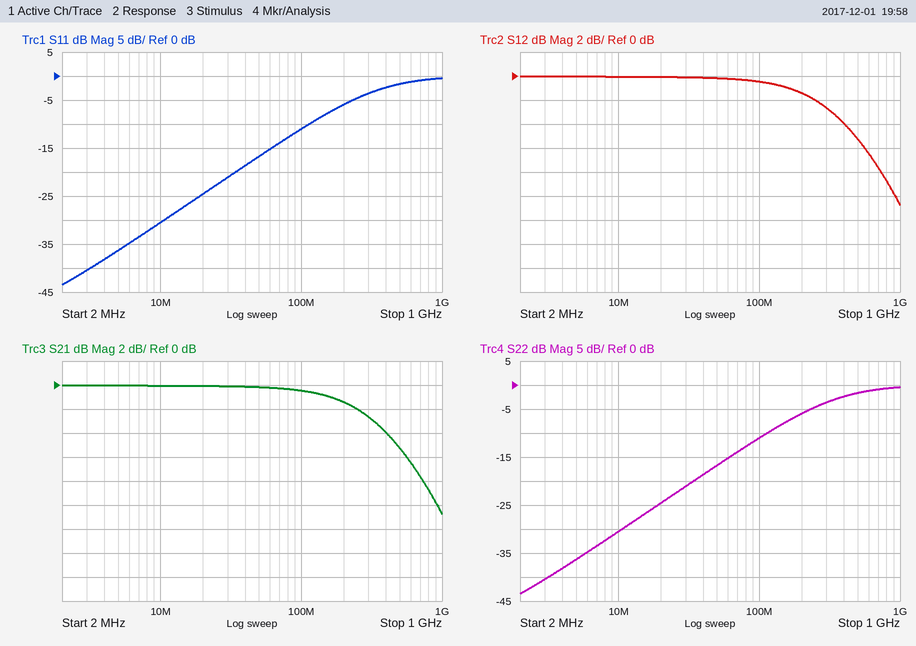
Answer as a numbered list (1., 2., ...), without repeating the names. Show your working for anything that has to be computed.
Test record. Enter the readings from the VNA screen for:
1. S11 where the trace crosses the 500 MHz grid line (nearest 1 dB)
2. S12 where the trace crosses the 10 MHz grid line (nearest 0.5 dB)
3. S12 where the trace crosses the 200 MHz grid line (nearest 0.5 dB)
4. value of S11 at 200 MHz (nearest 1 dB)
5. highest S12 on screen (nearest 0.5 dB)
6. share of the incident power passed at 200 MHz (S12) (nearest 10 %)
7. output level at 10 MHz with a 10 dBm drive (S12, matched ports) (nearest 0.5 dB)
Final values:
1. -2 dB
2. 0.0 dB
3. -1.5 dB
4. -6 dB
5. 0.0 dB
6. 10^(-1.5/10) ≈ 70.8 %, so 70 % to the nearest 10 %
7. 10 dBm + (0.0 dB) = 10.0 dBm
